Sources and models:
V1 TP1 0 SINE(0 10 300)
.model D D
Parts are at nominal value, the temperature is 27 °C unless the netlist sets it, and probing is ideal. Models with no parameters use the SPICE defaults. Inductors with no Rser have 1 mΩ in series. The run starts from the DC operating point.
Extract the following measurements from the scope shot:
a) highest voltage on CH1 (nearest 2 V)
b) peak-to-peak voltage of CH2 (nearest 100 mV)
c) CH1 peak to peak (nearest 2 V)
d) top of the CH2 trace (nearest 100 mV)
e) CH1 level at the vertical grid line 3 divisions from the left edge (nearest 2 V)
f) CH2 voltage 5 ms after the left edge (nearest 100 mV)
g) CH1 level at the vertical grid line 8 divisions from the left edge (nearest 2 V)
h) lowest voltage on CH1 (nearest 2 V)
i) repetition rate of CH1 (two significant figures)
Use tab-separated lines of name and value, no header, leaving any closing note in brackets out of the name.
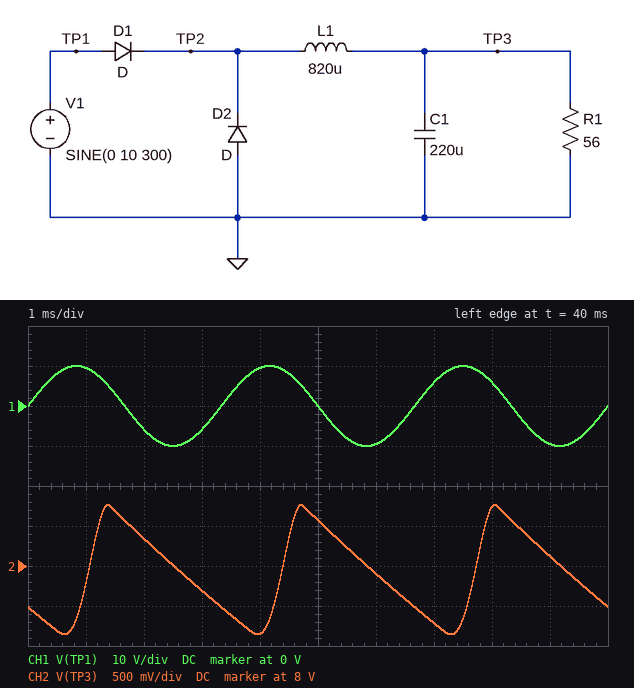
highest voltage on CH1	10 V
peak-to-peak voltage of CH2	1.6 V
CH1 peak to peak	20 V
top of the CH2 trace	8.8 V
CH1 level at the vertical grid line 3 divisions from the left edge	-6 V
CH2 voltage 5 ms after the left edge	8.6 V
CH1 level at the vertical grid line 8 divisions from the left edge	6 V
lowest voltage on CH1	-10 V
repetition rate of CH1	300 Hz
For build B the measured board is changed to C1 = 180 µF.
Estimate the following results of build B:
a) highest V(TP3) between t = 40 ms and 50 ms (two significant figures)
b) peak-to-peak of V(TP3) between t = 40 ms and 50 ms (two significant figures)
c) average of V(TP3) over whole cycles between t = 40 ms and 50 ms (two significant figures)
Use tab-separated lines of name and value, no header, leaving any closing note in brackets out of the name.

highest V(TP3) between t = 40 ms and 50 ms	9.0 V
peak-to-peak of V(TP3) between t = 40 ms and 50 ms	2.0 V
average of V(TP3) over whole cycles between t = 40 ms and 50 ms	8.0 V
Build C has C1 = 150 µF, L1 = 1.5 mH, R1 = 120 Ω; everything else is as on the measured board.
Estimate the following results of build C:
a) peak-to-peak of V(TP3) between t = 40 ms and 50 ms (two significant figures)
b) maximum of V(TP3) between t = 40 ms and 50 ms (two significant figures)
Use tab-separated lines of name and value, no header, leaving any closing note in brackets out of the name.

peak-to-peak of V(TP3) between t = 40 ms and 50 ms	1.1 V
maximum of V(TP3) between t = 40 ms and 50 ms	8.5 V
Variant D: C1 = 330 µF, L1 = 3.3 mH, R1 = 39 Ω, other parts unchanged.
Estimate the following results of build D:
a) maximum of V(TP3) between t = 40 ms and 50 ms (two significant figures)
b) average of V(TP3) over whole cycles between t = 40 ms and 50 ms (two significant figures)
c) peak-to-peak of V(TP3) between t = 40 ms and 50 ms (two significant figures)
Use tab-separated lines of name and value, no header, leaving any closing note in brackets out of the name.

maximum of V(TP3) between t = 40 ms and 50 ms	6.5 V
average of V(TP3) over whole cycles between t = 40 ms and 50 ms	6.0 V
peak-to-peak of V(TP3) between t = 40 ms and 50 ms	1.0 V
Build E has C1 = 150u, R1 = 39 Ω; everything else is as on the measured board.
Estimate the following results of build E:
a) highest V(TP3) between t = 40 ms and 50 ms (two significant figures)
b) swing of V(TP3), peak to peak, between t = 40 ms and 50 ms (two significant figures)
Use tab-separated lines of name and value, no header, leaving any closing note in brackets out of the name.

highest V(TP3) between t = 40 ms and 50 ms	9.7 V
swing of V(TP3), peak to peak, between t = 40 ms and 50 ms	3.3 V
